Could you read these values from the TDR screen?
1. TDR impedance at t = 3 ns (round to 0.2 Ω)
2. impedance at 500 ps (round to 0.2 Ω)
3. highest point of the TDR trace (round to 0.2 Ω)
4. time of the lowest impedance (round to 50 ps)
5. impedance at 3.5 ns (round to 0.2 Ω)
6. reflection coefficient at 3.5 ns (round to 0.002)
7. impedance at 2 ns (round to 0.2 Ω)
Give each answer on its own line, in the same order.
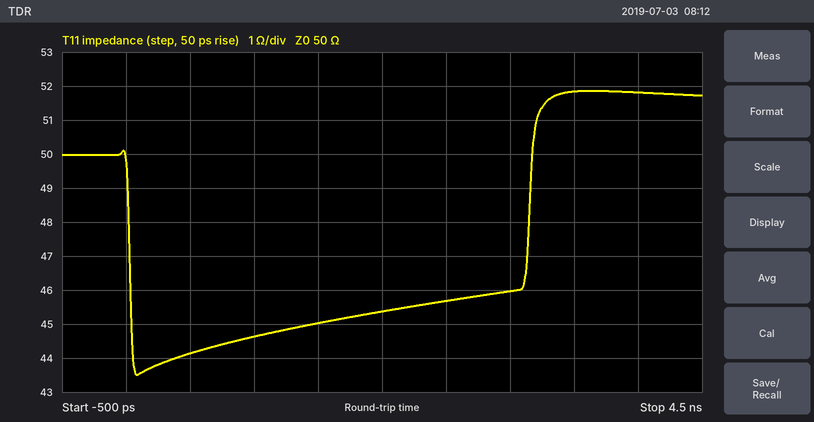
46.0 Ω
44.2 Ω
51.8 Ω
100 ps
51.8 Ω
+0.018
45.4 Ω
